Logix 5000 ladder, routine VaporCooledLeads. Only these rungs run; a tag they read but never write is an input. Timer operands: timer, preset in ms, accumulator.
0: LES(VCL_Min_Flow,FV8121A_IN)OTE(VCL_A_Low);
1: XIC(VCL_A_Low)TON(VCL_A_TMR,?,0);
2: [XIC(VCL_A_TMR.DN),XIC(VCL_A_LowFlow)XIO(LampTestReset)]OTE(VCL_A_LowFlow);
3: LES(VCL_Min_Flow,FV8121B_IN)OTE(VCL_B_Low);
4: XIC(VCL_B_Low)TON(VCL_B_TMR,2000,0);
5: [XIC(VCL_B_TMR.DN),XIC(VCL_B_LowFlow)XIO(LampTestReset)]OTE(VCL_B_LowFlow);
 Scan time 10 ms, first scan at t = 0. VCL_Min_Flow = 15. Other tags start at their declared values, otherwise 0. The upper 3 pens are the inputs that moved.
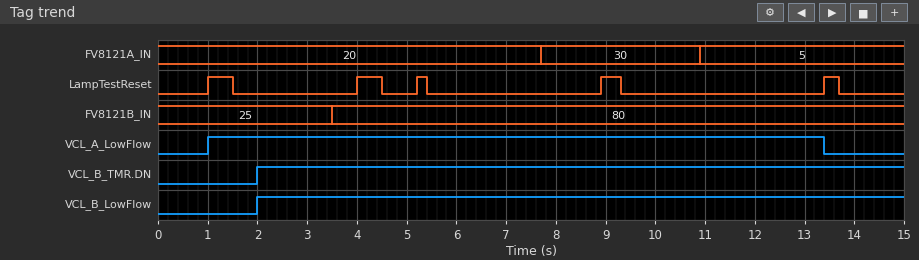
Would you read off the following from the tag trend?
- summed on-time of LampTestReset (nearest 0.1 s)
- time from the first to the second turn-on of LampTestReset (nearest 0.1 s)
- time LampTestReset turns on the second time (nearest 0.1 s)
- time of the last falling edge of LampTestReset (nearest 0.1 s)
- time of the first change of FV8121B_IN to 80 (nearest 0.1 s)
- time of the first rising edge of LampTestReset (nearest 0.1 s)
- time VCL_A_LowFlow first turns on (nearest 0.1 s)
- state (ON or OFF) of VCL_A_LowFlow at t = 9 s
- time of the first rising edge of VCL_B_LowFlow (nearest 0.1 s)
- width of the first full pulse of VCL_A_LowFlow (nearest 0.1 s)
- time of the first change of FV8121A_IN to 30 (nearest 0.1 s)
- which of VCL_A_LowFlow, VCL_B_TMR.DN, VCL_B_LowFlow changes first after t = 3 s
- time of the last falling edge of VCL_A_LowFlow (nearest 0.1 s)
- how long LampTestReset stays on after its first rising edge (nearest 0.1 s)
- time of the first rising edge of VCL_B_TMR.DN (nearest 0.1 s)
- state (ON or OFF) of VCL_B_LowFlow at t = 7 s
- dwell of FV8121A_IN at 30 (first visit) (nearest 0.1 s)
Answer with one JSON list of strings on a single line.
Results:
["1.9 s", "3.0 s", "4.0 s", "13.7 s", "3.5 s", "1.0 s", "1.0 s", "ON", "2.0 s", "12.4 s", "7.7 s", "VCL_A_LowFlow", "13.4 s", "0.5 s", "2.0 s", "ON", "3.2 s"]
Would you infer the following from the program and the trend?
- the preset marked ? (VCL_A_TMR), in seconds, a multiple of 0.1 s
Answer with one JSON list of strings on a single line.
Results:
["1.0 s"]
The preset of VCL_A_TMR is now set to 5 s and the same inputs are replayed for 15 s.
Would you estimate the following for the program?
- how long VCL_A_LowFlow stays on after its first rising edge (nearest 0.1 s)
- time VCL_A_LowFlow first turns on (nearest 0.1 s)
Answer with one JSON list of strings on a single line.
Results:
["8.4 s", "5.0 s"]
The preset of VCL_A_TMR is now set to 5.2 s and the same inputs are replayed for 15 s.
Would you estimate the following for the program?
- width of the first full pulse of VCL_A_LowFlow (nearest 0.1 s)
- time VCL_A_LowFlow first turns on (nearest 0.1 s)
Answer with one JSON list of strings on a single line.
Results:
["8.2 s", "5.2 s"]
